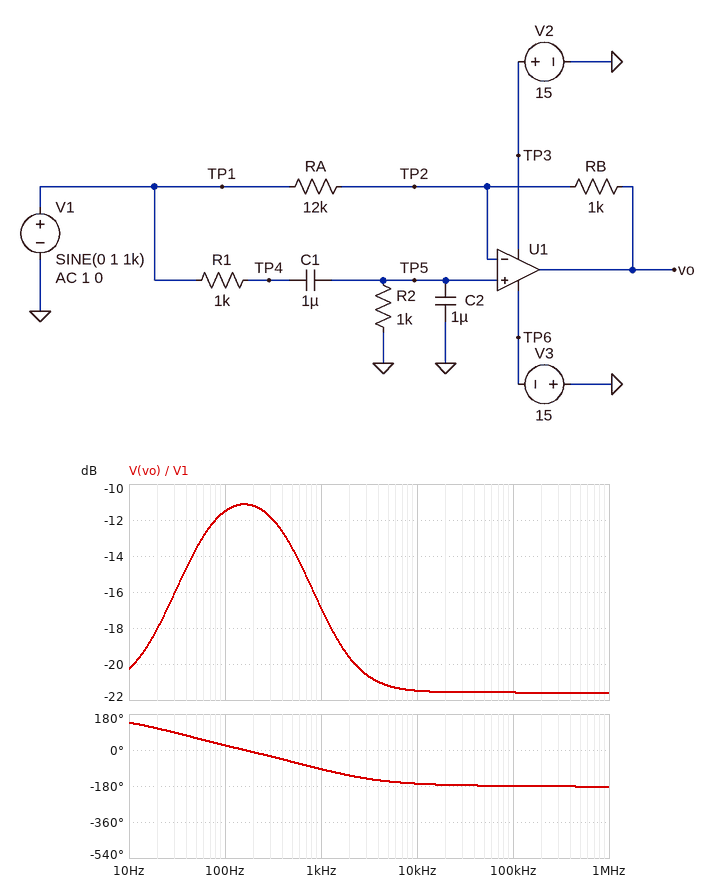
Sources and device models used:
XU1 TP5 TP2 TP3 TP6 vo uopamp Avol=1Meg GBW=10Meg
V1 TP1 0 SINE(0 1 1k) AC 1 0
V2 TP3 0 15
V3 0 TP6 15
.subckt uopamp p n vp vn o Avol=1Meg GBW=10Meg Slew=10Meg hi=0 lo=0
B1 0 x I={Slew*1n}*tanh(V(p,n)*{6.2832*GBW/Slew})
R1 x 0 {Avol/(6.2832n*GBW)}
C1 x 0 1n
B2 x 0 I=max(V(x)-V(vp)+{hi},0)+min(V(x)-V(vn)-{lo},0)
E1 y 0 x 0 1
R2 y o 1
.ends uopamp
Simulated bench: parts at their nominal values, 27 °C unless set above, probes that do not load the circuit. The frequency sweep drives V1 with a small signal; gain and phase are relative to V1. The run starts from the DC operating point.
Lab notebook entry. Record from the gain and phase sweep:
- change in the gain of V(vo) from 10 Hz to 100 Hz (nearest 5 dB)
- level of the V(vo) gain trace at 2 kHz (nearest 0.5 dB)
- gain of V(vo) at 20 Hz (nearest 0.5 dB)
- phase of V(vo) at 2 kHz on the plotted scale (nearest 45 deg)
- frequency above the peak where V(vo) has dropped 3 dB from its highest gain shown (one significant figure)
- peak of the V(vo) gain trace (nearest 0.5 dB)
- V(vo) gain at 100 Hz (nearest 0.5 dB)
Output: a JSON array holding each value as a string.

["10 dB", "-19.5 dB", "-18.0 dB", "-135 deg", "600 Hz", "-11.0 dB", "-11.5 dB"]
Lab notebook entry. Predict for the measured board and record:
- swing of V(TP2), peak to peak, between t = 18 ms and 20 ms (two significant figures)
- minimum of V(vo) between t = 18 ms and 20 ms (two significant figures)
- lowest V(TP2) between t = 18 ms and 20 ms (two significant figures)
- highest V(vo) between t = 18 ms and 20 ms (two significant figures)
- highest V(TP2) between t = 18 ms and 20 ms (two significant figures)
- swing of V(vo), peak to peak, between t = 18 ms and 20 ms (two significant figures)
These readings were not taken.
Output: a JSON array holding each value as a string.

["290 mV", "-140 mV", "-150 mV", "140 mV", "150 mV", "290 mV"]
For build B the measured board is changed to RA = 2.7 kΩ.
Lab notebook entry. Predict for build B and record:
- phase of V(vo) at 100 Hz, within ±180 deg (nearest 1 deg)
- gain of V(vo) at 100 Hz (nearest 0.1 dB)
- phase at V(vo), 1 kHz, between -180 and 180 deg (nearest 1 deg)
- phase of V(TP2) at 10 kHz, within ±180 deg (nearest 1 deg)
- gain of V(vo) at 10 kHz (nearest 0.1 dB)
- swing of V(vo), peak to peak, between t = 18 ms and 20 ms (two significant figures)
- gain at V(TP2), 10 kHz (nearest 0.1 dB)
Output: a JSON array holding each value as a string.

["72 deg", "-17.1 dB", "-147 deg", "-87 deg", "-8.6 dB", "670 mV", "-36.2 dB"]
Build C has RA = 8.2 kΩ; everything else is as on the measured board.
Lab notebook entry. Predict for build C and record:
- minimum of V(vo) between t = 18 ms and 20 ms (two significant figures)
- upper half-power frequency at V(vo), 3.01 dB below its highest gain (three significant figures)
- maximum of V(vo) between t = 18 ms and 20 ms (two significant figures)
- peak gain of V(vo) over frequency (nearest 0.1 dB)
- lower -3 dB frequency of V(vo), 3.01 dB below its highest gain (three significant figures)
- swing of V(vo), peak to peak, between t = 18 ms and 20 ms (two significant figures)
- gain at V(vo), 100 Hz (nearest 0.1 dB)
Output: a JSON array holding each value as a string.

["-160 mV", "691 Hz", "160 mV", "-12.0 dB", "36.6 Hz", "310 mV", "-12.3 dB"]
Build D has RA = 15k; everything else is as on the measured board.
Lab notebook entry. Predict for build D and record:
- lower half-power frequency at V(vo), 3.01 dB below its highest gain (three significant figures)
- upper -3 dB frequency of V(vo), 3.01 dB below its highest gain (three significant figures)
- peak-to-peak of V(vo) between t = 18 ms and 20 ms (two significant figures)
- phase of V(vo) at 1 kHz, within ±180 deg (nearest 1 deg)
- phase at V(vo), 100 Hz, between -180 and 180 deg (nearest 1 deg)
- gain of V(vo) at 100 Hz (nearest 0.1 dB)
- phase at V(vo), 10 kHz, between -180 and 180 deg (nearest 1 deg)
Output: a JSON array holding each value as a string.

["46.0 Hz", "551 Hz", "280 mV", "-89 deg", "22 deg", "-11.2 dB", "-166 deg"]
